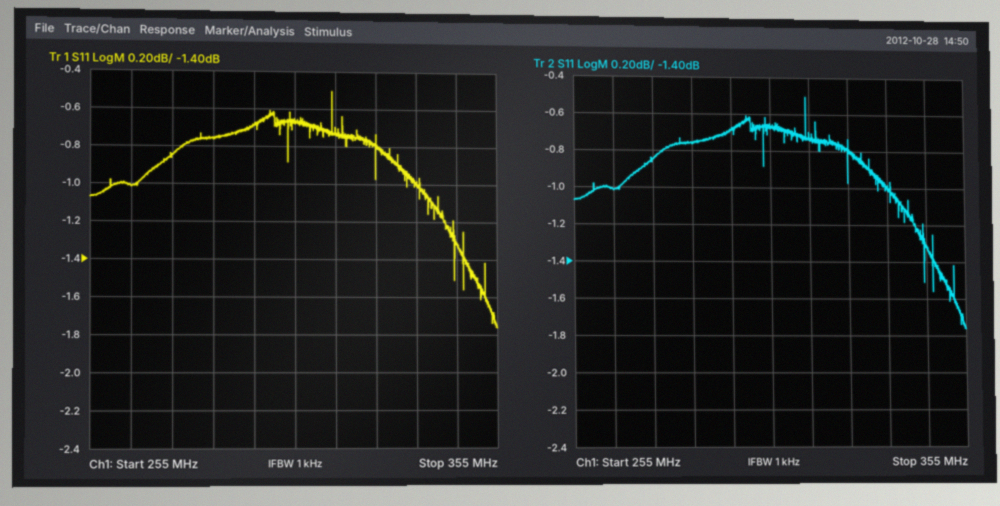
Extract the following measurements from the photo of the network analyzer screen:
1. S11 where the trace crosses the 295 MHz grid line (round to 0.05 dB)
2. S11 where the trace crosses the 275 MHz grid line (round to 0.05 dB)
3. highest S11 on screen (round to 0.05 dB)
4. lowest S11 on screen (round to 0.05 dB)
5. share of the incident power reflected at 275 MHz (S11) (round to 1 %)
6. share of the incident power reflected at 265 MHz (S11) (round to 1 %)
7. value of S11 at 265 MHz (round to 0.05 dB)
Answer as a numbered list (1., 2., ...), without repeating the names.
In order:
1. -0.70 dB
2. -0.85 dB
3. -0.50 dB
4. -1.75 dB
5. 82 %
6. 79 %
7. -1.00 dB
